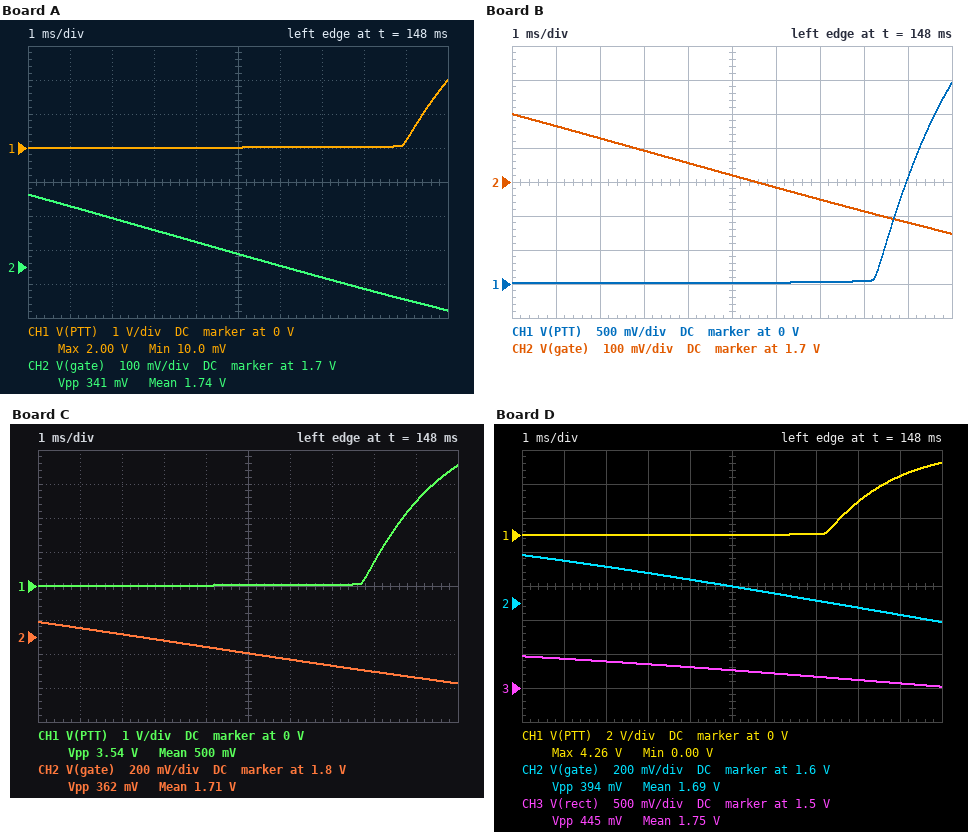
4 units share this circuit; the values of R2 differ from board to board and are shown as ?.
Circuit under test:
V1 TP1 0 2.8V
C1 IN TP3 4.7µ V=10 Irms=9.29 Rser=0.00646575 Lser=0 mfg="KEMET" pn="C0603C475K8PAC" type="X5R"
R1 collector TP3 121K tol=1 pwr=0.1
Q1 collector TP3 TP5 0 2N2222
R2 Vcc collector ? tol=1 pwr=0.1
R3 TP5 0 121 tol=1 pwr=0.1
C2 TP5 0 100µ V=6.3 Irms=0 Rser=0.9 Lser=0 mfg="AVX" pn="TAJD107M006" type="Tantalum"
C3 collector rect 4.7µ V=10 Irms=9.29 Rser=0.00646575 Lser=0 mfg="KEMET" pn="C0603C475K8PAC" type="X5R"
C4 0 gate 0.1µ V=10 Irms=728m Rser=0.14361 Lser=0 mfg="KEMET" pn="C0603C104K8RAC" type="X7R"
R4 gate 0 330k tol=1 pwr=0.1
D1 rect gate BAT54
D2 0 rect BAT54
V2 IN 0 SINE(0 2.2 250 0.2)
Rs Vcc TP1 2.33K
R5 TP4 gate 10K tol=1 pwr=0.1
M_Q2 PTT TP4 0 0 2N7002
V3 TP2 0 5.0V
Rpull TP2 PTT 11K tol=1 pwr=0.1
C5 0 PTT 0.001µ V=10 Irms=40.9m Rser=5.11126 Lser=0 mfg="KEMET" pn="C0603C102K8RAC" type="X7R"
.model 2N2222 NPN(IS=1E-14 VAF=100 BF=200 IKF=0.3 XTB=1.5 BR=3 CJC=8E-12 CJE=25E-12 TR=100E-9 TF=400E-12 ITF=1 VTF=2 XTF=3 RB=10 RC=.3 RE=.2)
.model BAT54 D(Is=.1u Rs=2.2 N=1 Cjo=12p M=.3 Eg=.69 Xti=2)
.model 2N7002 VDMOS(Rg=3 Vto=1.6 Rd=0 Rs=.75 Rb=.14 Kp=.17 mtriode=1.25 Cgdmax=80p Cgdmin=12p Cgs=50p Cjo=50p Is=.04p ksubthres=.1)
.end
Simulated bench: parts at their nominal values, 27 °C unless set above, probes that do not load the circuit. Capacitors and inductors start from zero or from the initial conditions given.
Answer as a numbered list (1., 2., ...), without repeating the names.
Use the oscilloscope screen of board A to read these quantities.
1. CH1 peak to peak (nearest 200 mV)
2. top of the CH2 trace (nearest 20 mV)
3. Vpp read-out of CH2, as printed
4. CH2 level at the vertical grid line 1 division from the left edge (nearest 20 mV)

1. 2.0 V
2. 1.92 V
3. 341 mV
4. 1.88 V
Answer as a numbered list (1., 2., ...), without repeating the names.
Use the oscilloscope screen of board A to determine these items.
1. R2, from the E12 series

1. 1.2 kΩ
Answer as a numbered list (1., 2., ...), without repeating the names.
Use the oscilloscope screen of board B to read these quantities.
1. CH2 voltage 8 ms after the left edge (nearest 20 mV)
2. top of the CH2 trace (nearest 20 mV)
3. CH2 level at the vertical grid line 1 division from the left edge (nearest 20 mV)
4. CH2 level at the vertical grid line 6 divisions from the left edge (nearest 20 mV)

1. 1.62 V
2. 1.90 V
3. 1.86 V
4. 1.68 V
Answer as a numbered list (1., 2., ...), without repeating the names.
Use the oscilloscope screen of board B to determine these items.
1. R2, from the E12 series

1. 1.5 kΩ
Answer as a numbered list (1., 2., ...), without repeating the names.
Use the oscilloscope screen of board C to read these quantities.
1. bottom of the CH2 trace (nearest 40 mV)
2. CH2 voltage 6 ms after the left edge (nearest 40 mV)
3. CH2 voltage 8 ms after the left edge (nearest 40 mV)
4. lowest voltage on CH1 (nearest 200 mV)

1. 1.52 V
2. 1.68 V
3. 1.60 V
4. 0 V
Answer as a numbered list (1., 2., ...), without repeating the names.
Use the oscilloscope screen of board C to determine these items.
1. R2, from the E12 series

1. 1.8 kΩ
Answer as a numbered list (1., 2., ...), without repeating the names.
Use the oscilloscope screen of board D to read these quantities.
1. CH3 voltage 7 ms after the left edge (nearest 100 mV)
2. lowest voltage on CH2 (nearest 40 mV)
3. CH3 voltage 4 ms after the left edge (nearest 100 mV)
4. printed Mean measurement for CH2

1. 1.7 V
2. 1.48 V
3. 1.8 V
4. 1.69 V
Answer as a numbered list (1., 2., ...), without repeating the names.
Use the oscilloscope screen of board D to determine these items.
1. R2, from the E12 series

1. 8.2 kΩ
